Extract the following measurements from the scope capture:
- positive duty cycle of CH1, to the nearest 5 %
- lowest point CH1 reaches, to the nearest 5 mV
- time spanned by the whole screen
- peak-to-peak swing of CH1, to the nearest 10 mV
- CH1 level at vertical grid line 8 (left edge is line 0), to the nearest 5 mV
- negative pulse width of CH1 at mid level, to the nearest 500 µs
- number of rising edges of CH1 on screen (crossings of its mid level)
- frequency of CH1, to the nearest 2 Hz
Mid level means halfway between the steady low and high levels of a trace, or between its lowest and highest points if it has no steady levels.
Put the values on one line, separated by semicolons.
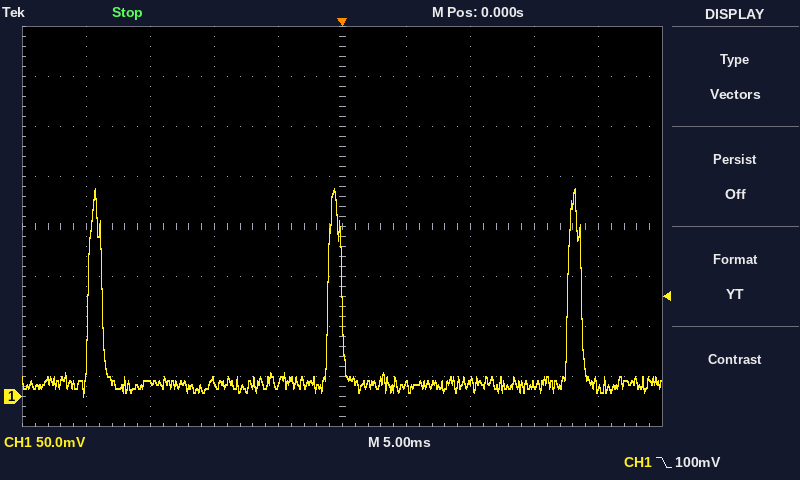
5 %; 0 mV; 50 ms; 210 mV; 10 mV; 17.5 ms; 3; 54 Hz
